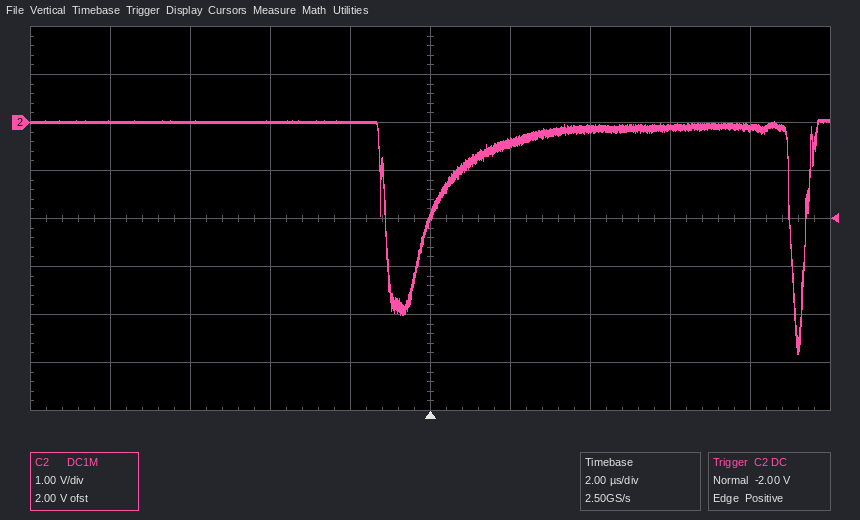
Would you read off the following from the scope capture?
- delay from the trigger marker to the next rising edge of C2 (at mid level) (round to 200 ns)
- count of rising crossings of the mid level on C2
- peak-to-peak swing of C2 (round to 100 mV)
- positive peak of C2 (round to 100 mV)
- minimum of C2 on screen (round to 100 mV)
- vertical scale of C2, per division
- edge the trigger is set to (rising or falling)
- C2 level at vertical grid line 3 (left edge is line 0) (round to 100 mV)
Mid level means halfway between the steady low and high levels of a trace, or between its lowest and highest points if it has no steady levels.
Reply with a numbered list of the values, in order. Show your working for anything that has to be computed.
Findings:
1. 9.4 µs
2. 2
3. 100 mV − (-4.8 V) = 4.9 V
4. 100 mV
5. -4.8 V
6. 1 V
7. rising
8. 0.0 V
